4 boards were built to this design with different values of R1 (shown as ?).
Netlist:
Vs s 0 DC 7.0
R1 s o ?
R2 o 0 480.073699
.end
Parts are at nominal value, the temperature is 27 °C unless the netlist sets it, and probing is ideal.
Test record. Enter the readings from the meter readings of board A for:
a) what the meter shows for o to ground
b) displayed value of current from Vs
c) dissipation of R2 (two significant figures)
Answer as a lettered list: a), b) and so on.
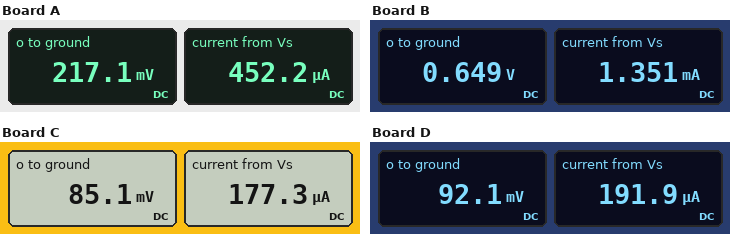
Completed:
a) 217.1 mV
b) 452.2 µA
c) 98 µW
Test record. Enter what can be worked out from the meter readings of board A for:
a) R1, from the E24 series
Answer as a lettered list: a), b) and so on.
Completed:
a) 15 kΩ
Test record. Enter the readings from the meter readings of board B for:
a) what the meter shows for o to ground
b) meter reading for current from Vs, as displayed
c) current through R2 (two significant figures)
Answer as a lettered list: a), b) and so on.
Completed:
a) 0.649 V
b) 1.351 mA
c) 1.4 mA
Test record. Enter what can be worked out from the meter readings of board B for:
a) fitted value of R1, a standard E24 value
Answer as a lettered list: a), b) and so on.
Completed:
a) 4.7 kΩ
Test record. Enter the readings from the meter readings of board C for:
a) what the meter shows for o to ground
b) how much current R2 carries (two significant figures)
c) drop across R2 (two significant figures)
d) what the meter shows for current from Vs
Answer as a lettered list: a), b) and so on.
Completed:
a) 85.1 mV
b) 180 µA
c) 85 mV
d) 177.3 µA
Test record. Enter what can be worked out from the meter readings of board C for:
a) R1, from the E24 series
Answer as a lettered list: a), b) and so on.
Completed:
a) 39 kΩ
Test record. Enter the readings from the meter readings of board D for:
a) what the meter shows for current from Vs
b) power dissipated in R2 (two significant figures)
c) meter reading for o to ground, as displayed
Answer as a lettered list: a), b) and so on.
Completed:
a) 191.9 µA
b) 18 µW
c) 92.1 mV
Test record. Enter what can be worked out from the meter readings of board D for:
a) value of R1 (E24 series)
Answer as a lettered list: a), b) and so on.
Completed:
a) 36 kΩ
